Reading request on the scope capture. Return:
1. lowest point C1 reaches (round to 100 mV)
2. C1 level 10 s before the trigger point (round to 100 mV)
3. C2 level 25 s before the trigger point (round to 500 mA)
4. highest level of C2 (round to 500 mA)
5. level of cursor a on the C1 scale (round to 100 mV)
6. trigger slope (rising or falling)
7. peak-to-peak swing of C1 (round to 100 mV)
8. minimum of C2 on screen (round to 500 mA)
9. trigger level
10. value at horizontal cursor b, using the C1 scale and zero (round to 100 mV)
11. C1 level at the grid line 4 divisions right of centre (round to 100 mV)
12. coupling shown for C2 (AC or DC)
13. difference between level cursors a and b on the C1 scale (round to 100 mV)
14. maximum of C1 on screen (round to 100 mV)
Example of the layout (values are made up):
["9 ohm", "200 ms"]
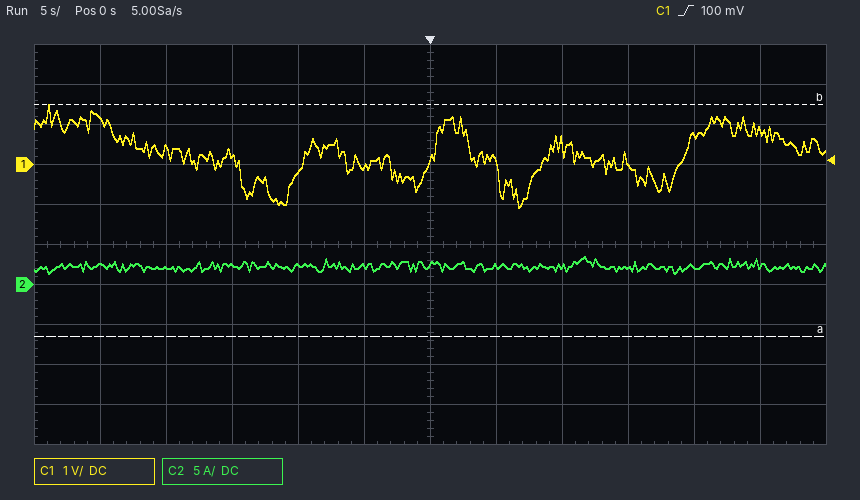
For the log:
["-1.1 V", "-200 mV", "2.5 A", "3.5 A", "-4.3 V", "rising", "2.6 V", "1.5 A", "100 mV", "1.5 V", "700 mV", "DC", "5.8 V", "1.5 V"]
